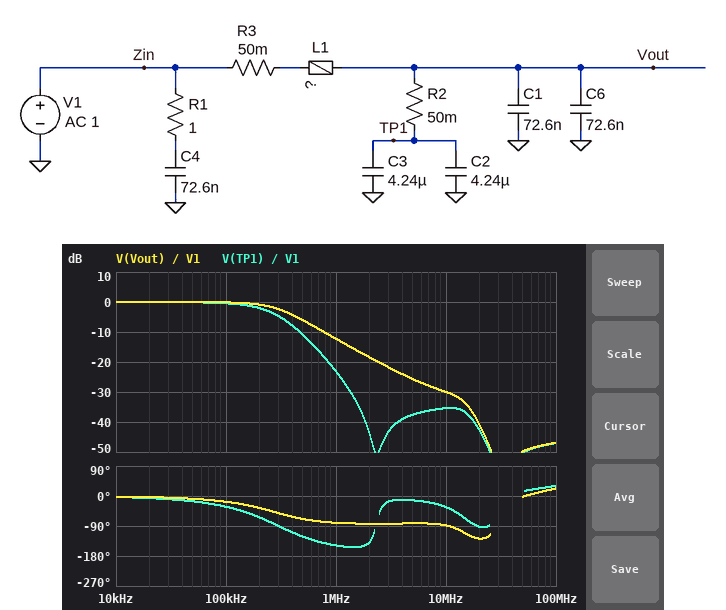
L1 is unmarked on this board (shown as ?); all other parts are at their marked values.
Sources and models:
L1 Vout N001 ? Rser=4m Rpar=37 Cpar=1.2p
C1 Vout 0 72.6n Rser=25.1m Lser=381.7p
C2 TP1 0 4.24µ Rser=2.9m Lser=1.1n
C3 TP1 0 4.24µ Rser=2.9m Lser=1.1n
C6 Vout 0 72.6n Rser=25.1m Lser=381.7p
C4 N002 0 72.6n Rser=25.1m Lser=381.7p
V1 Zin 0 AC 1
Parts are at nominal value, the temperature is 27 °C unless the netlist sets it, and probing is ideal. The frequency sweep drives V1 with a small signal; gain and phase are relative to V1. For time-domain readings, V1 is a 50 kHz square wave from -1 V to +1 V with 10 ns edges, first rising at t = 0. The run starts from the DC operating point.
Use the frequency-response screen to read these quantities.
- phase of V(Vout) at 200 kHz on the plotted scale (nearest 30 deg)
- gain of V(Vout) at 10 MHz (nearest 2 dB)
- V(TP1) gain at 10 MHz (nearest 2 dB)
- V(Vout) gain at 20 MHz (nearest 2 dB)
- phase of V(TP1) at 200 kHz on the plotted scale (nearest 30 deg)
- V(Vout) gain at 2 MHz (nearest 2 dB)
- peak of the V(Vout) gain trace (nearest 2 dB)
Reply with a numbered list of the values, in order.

1. -30 deg
2. -30 dB
3. -36 dB
4. -40 dB
5. -60 deg
6. -18 dB
7. 0 dB
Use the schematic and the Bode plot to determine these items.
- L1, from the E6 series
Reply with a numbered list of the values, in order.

1. 33 nH
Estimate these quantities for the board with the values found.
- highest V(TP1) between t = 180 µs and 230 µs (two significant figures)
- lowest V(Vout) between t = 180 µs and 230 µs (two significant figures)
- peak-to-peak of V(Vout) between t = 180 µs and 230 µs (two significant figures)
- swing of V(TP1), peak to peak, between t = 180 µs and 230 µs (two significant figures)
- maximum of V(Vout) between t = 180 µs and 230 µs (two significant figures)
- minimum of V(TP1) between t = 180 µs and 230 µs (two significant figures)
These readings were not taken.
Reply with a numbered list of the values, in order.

1. 1.0 V
2. -1.0 V
3. 2.1 V
4. 2.0 V
5. 1.0 V
6. -1.0 V
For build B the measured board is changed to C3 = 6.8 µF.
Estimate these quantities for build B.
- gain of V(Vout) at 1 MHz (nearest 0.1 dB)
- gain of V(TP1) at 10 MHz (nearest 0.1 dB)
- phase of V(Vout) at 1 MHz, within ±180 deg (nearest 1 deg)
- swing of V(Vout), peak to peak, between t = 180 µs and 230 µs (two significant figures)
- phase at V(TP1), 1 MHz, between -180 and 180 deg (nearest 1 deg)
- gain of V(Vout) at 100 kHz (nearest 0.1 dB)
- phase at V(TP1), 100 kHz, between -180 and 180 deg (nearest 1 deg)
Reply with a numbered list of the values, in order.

1. -12.6 dB
2. -35.3 dB
3. -76 deg
4. 2.0 V
5. -146 deg
6. -0.5 dB
7. -40 deg
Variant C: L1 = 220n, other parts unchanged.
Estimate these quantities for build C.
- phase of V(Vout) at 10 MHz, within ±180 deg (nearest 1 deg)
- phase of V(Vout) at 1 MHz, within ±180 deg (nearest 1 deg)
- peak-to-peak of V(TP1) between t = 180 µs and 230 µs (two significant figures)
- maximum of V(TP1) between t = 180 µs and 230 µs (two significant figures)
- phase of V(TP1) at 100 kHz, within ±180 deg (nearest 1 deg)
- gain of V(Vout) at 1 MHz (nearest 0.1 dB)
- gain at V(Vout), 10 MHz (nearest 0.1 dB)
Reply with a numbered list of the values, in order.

1. -74 deg
2. -103 deg
3. 3.2 V
4. 1.6 V
5. -66 deg
6. -28.3 dB
7. -45.9 dB
